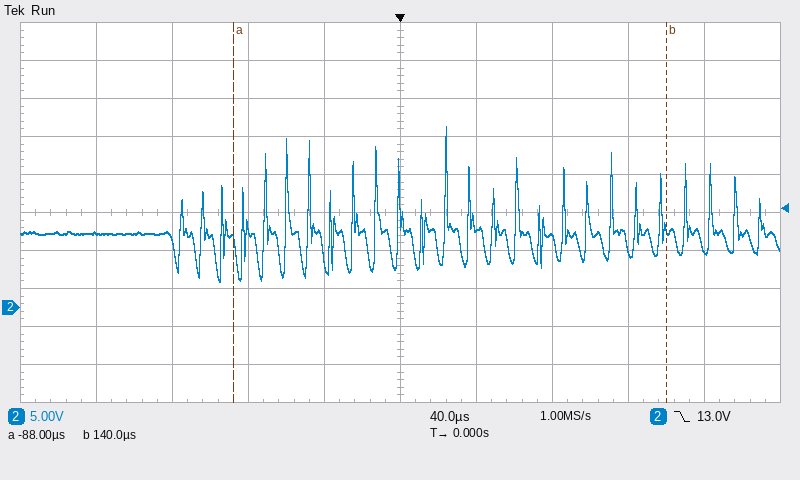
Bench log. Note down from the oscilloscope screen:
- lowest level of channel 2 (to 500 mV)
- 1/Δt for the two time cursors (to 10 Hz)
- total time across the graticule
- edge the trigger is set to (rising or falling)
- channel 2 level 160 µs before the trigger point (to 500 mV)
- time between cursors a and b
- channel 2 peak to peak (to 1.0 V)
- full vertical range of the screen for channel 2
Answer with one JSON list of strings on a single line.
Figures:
["3.5 V", "4.39 kHz", "400 µs", "falling", "10.0 V", "228 µs", "20.0 V", "50 V"]
